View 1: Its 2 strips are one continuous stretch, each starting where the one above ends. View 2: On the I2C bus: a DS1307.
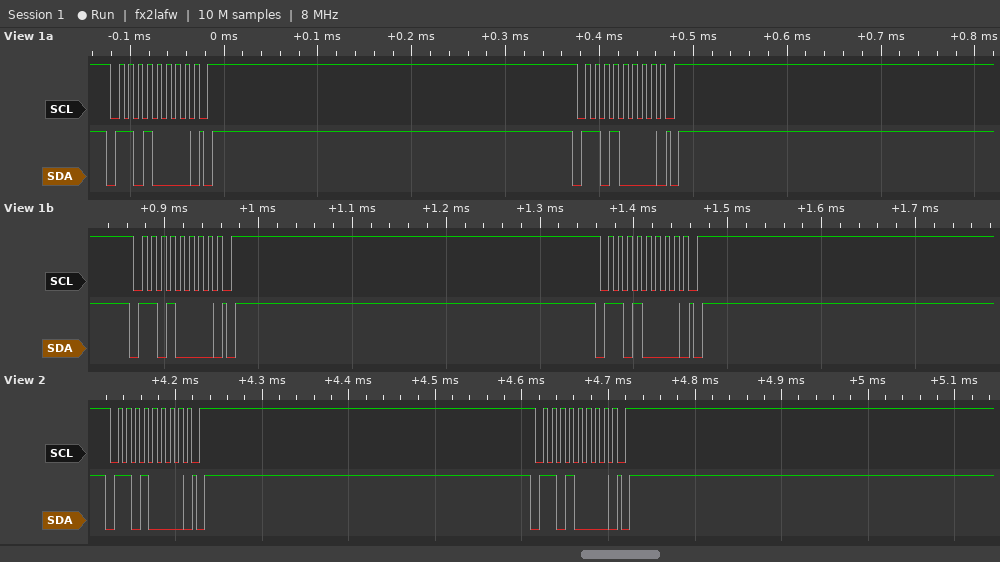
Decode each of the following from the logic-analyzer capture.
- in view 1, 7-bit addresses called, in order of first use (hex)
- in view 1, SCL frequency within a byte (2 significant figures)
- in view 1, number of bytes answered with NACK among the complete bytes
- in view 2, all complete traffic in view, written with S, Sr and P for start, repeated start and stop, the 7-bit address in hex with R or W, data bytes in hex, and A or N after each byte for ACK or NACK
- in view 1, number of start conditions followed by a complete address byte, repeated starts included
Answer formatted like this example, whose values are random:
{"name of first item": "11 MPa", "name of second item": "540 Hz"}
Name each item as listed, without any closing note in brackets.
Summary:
{"in view 1, 7-bit addresses called, in order of first use": "0x68", "in view 1, SCL frequency within a byte": "100 kHz", "in view 1, number of bytes answered with NACK among the complete bytes": "0", "in view 2, all complete traffic in view, written with S, Sr and P for start, repeated start and stop, the 7-bit address in hex with R or W, data bytes in hex, and A or N after each byte for ACK or NACK": "S 68W A P S 68W A P", "in view 1, number of start conditions followed by a complete address byte, repeated starts included": "4"}
